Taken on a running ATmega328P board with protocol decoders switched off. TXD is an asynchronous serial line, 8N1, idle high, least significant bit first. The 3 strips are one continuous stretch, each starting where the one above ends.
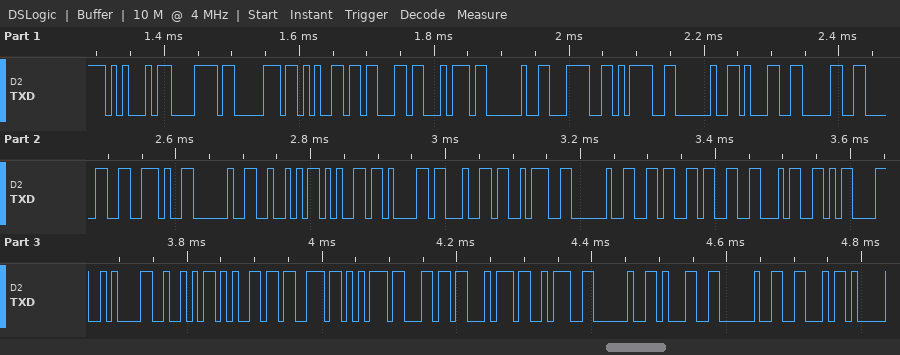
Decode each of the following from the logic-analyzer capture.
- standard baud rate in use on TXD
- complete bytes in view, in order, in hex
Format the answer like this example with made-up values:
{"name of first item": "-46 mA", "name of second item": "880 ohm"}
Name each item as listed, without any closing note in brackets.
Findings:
{"standard baud rate in use on TXD": "115200 baud", "complete bytes in view, in order, in hex": "45 78 70 65 63 74 20 3C 3D 20 31 30 30 2E 20 52 65 61 64 3A 20 36 33 34 0D 0A 52 65 73 75 6C 74 3A 20 31 20 46"}
